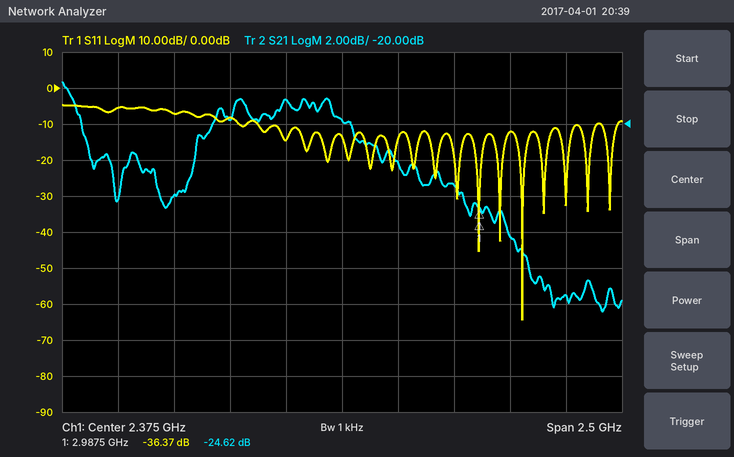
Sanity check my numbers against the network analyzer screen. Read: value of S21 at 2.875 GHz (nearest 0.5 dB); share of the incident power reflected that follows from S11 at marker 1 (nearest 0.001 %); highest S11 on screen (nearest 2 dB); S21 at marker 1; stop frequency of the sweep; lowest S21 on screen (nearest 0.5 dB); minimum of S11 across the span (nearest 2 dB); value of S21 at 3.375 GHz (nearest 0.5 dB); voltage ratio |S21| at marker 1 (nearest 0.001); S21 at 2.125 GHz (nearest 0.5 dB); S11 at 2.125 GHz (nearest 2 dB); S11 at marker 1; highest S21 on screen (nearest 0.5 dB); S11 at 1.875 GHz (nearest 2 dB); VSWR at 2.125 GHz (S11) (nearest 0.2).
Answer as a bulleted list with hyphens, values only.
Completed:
- -23.5 dB
- 0.023 %
- -4 dB
- -24.62 dB
- 3.625 GHz
- -30.5 dB
- -64 dB
- -29.5 dB
- 0.059
- -18.5 dB
- -14 dB
- -36.37 dB
- -17.5 dB
- -8 dB
- 1.4
